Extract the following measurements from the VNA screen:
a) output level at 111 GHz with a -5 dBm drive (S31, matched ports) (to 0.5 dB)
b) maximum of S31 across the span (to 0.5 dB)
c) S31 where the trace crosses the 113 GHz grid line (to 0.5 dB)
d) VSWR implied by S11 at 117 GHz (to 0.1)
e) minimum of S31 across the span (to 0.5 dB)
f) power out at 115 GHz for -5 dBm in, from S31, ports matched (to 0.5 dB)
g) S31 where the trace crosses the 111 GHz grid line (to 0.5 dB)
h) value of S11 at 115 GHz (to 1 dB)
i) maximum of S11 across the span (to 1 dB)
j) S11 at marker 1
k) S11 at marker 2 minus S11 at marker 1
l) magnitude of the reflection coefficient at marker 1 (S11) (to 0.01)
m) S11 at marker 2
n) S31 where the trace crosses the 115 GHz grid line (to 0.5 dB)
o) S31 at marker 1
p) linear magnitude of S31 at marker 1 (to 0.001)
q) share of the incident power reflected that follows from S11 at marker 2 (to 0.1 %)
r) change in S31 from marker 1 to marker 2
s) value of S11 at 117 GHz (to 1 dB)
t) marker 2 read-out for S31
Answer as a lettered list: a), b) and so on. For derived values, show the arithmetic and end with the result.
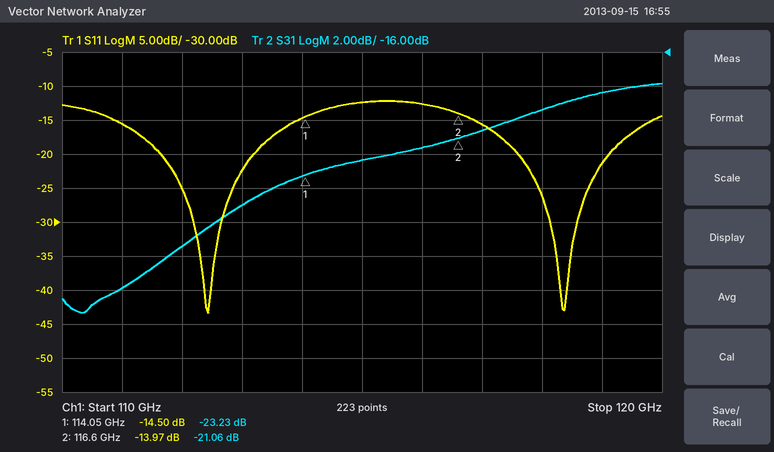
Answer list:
a) -5 dBm + (-30.0 dB) = -35.0 dBm
b) -18.0 dB
c) -25.0 dB
d) |Γ| = 10^(-16/20) = 0.1585; VSWR = (1 + 0.1585)/(1 − 0.1585) ≈ 1.4
e) -31.5 dB
f) -5 dBm + (-22.5 dB) = -27.5 dBm
g) -30.0 dB
h) -12 dB
i) -12 dB
j) -14.50 dB
k) -13.97 − (-14.5) = 0.53 dB
l) 10^(-14.5/20) ≈ 0.19
m) -13.97 dB
n) -22.5 dB
o) -23.23 dB
p) 10^(-23.23/20) ≈ 0.069
q) 10^(-13.97/10) ≈ 4.0 %
r) -21.06 − (-23.23) = 2.17 dB
s) -16 dB
t) -21.06 dB
